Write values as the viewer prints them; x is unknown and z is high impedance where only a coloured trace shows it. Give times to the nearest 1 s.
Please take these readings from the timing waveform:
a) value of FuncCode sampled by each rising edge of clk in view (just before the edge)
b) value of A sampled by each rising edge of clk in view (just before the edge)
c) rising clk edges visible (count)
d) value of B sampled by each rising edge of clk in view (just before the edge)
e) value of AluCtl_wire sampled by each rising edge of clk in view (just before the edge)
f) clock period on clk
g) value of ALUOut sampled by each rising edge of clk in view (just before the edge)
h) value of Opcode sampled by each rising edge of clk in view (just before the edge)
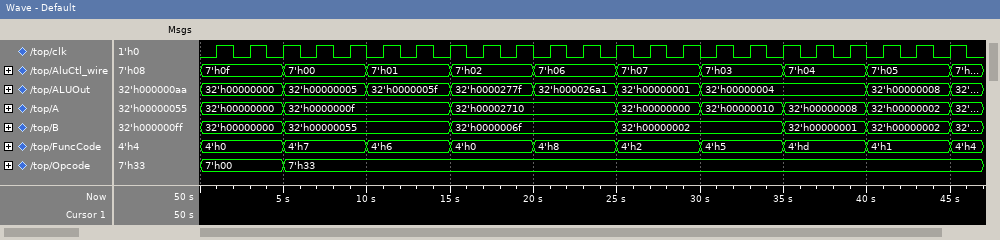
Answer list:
4'h0, 4'h0, 4'h0, 4'h7, 4'h7, 4'h6, 4'h6, 4'h6, 4'h0, 4'h0, 4'h8, 4'h8, 4'h8, 4'h2, 4'h2, 4'h5, 4'h5, 4'h5, 4'hd, 4'hd, 4'h1, 4'h1, 4'h1
32'h00000000, 32'h00000000, 32'h00000000, 32'h0000000f, 32'h0000000f, 32'h0000000f, 32'h0000000f, 32'h0000000f, 32'h00002710, 32'h00002710, 32'h00002710, 32'h00002710, 32'h00002710, 32'h00000000, 32'h00000000, 32'h00000010, 32'h00000010, 32'h00000010, 32'h00000008, 32'h00000008, 32'h00000002, 32'h00000002, 32'h00000002
23
32'h00000000, 32'h00000000, 32'h00000000, 32'h00000055, 32'h00000055, 32'h00000055, 32'h00000055, 32'h00000055, 32'h0000006f, 32'h0000006f, 32'h0000006f, 32'h0000006f, 32'h0000006f, 32'h00000002, 32'h00000002, 32'h00000002, 32'h00000002, 32'h00000002, 32'h00000001, 32'h00000001, 32'h00000002, 32'h00000002, 32'h00000002
7'h0f, 7'h0f, 7'h0f, 7'h00, 7'h00, 7'h01, 7'h01, 7'h01, 7'h02, 7'h02, 7'h06, 7'h06, 7'h06, 7'h07, 7'h07, 7'h03, 7'h03, 7'h03, 7'h04, 7'h04, 7'h05, 7'h05, 7'h05
2 s
32'h00000000, 32'h00000000, 32'h00000000, 32'h00000005, 32'h00000005, 32'h0000005f, 32'h0000005f, 32'h0000005f, 32'h0000277f, 32'h0000277f, 32'h000026a1, 32'h000026a1, 32'h000026a1, 32'h00000001, 32'h00000001, 32'h00000004, 32'h00000004, 32'h00000004, 32'h00000004, 32'h00000004, 32'h00000008, 32'h00000008, 32'h00000008
7'h00, 7'h00, 7'h00, 7'h33, 7'h33, 7'h33, 7'h33, 7'h33, 7'h33, 7'h33, 7'h33, 7'h33, 7'h33, 7'h33, 7'h33, 7'h33, 7'h33, 7'h33, 7'h33, 7'h33, 7'h33, 7'h33, 7'h33
